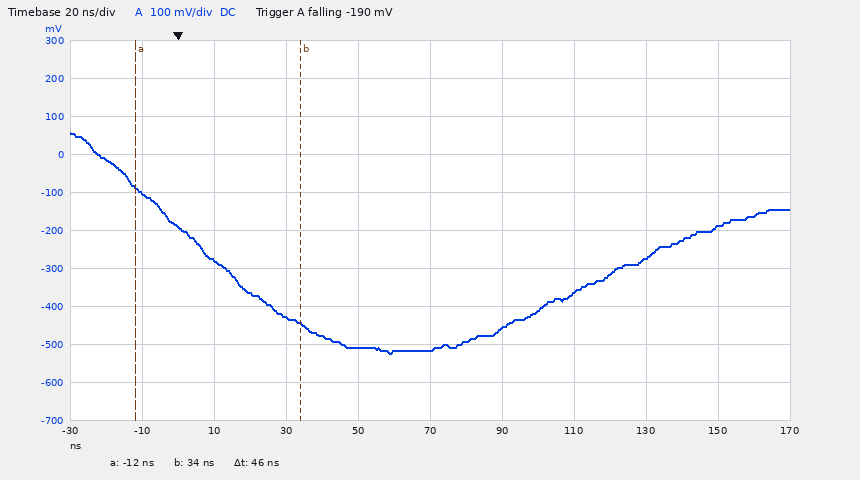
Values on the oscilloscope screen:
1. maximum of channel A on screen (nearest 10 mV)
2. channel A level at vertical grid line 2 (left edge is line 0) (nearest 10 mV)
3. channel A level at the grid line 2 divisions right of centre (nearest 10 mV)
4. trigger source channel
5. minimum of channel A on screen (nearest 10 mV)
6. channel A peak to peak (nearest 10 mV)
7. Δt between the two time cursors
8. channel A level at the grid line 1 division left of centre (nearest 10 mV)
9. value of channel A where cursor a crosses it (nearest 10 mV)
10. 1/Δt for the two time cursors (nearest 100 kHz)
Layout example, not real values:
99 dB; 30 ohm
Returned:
60 mV; -280 mV; -360 mV; channel A; -520 mV; 580 mV; 46 ns; -510 mV; -90 mV; 21.7 MHz
